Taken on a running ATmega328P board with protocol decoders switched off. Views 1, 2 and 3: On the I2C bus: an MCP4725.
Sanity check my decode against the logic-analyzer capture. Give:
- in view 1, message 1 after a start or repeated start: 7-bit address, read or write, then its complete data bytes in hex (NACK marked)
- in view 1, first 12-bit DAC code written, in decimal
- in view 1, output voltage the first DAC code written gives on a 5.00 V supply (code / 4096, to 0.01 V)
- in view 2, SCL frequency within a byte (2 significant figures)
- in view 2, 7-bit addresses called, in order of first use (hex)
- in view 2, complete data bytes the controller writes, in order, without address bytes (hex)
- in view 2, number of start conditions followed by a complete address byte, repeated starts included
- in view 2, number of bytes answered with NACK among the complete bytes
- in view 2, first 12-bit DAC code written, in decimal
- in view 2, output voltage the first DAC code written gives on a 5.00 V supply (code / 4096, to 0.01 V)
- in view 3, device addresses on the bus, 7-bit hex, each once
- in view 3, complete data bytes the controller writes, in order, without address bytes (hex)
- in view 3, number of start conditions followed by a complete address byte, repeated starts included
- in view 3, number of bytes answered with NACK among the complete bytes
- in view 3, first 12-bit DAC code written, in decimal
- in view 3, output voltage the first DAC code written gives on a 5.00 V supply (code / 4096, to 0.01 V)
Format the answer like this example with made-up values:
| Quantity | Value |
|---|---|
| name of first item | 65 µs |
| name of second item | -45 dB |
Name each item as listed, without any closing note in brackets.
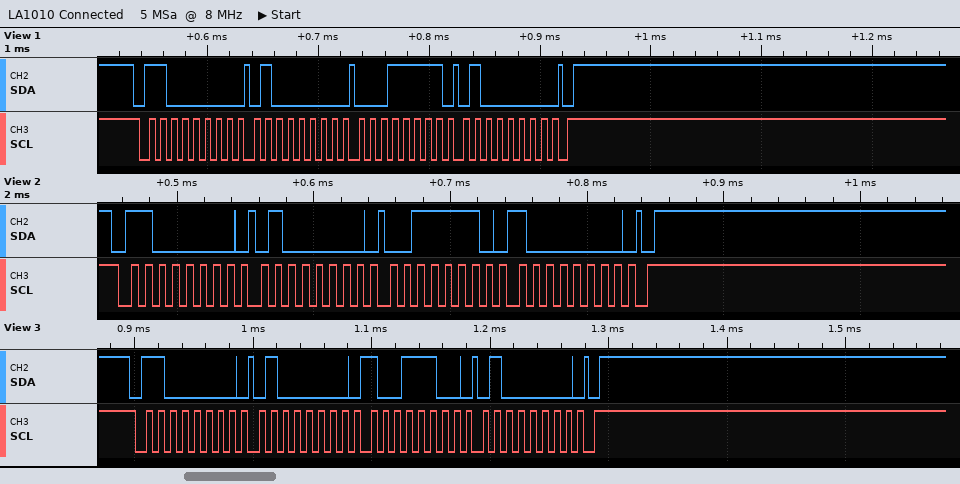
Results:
| Quantity | Value |
|---|---|
| in view 1, message 1 after a start or repeated start: 7-bit address, read or write, then its complete data bytes in hex | 0x60 write: 40 1F 40 |
| in view 1, first 12-bit DAC code written, in decimal | 500 |
| in view 1, output voltage the first DAC code written gives on a 5.00 V supply | 0.61 V |
| in view 2, SCL frequency within a byte | 100 kHz |
| in view 2, 7-bit addresses called, in order of first use | 0x60 |
| in view 2, complete data bytes the controller writes, in order, without address bytes | 40 3E 80 |
| in view 2, number of start conditions followed by a complete address byte, repeated starts included | 1 |
| in view 2, number of bytes answered with NACK among the complete bytes | 0 |
| in view 2, first 12-bit DAC code written, in decimal | 1000 |
| in view 2, output voltage the first DAC code written gives on a 5.00 V supply | 1.22 V |
| in view 3, device addresses on the bus, 7-bit hex, each once | 0x60 |
| in view 3, complete data bytes the controller writes, in order, without address bytes | 40 9C 40 |
| in view 3, number of start conditions followed by a complete address byte, repeated starts included | 1 |
| in view 3, number of bytes answered with NACK among the complete bytes | 0 |
| in view 3, first 12-bit DAC code written, in decimal | 2500 |
| in view 3, output voltage the first DAC code written gives on a 5.00 V supply | 3.05 V |
